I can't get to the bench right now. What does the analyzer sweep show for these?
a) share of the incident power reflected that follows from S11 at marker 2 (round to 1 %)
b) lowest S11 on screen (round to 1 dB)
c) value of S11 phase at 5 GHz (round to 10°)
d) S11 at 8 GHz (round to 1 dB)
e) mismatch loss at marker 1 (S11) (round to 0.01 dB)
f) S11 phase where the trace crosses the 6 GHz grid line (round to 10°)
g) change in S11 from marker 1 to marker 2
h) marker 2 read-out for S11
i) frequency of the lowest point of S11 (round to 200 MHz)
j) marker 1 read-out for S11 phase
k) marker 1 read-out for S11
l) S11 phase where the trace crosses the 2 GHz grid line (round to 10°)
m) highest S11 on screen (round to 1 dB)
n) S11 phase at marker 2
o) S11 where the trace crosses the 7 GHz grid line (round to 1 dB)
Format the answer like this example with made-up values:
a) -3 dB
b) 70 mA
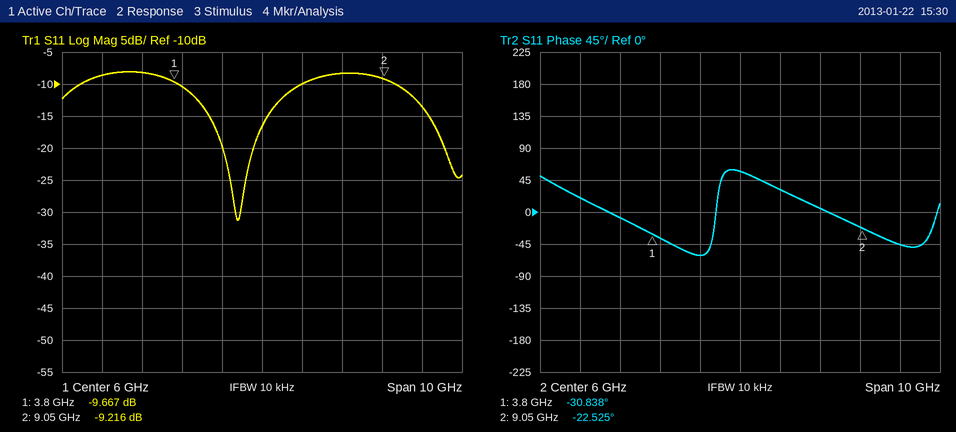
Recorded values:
a) 12 %
b) -31 dB
c) -60°
d) -8 dB
e) 0.50 dB
f) 60°
g) 0.451 dB
h) -9.216 dB
i) 5.4 GHz
j) -30.838°
k) -9.667 dB
l) 20°
m) -8 dB
n) -22.525°
o) -10 dB
